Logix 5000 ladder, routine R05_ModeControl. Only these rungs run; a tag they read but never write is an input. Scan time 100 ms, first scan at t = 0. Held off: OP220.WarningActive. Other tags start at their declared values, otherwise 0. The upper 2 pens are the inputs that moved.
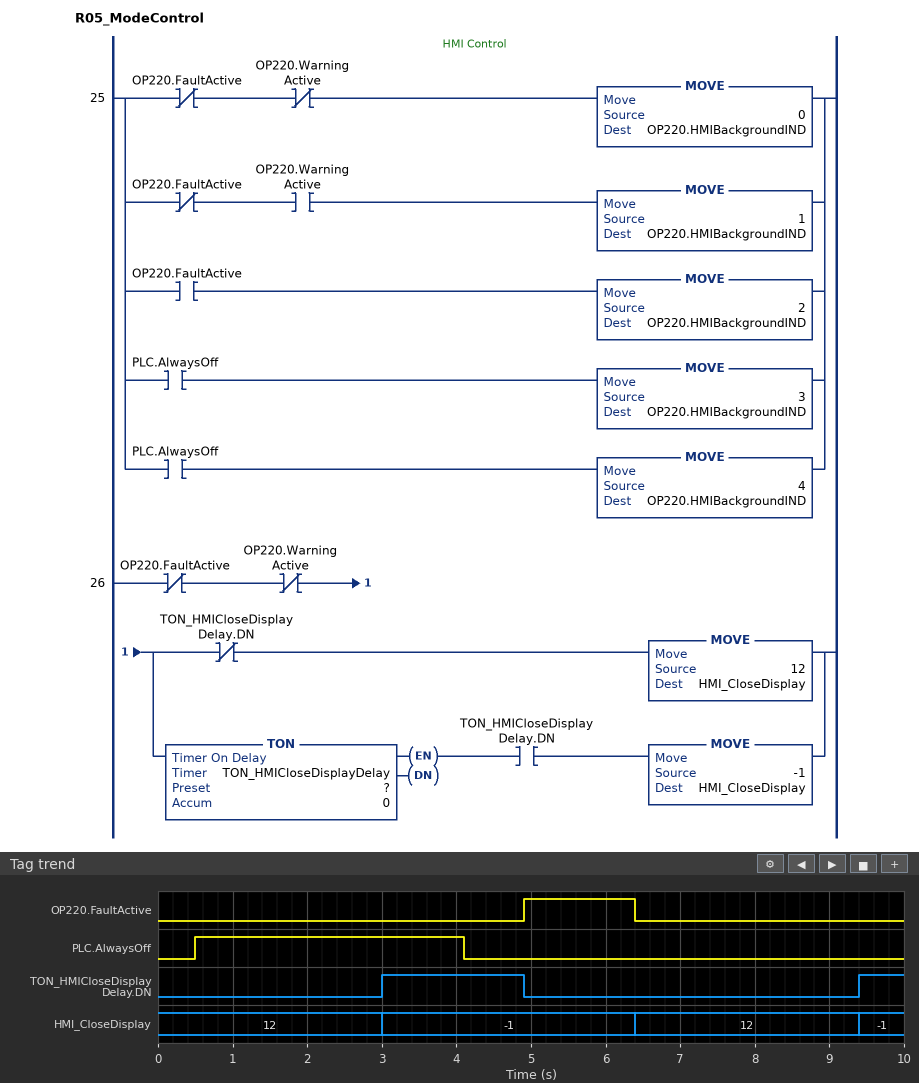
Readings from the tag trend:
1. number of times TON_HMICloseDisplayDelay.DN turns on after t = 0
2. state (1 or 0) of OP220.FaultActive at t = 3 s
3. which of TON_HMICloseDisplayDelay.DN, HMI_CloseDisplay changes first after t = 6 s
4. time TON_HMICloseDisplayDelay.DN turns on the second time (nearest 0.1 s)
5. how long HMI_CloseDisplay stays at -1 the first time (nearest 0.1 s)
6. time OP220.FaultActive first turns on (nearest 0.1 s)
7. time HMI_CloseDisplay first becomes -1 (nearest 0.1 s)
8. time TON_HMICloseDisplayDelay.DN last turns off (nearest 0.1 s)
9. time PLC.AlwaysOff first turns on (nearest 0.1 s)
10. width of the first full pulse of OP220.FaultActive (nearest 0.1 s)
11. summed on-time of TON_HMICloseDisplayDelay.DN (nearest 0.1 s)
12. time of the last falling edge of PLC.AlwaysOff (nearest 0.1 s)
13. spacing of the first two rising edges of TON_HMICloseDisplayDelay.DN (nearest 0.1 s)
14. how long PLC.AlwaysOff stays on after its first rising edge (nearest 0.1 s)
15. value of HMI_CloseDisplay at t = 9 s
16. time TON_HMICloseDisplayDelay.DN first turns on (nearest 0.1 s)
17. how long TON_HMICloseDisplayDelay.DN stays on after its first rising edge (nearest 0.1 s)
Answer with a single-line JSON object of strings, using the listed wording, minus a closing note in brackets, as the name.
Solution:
{"number of times TON_HMICloseDisplayDelay.DN turns on after t = 0": "2", "state (1 or 0) of OP220.FaultActive at t = 3 s": "0", "which of TON_HMICloseDisplayDelay.DN, HMI_CloseDisplay changes first after t = 6 s": "HMI_CloseDisplay", "time TON_HMICloseDisplayDelay.DN turns on the second time": "9.4 s", "how long HMI_CloseDisplay stays at -1 the first time": "3.4 s", "time OP220.FaultActive first turns on": "4.9 s", "time HMI_CloseDisplay first becomes -1": "3.0 s", "time TON_HMICloseDisplayDelay.DN last turns off": "4.9 s", "time PLC.AlwaysOff first turns on": "0.5 s", "width of the first full pulse of OP220.FaultActive": "1.5 s", "summed on-time of TON_HMICloseDisplayDelay.DN": "2.5 s", "time of the last falling edge of PLC.AlwaysOff": "4.1 s", "spacing of the first two rising edges of TON_HMICloseDisplayDelay.DN": "6.4 s", "how long PLC.AlwaysOff stays on after its first rising edge": "3.6 s", "value of HMI_CloseDisplay at t = 9 s": "12", "time TON_HMICloseDisplayDelay.DN first turns on": "3.0 s", "how long TON_HMICloseDisplayDelay.DN stays on after its first rising edge": "1.9 s"}
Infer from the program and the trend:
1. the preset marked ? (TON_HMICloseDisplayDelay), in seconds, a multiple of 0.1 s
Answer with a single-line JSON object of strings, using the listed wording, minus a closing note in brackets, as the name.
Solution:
{"the preset marked ? (TON_HMICloseDisplayDelay), in seconds, a multiple of 0.1 s": "3.0 s"}
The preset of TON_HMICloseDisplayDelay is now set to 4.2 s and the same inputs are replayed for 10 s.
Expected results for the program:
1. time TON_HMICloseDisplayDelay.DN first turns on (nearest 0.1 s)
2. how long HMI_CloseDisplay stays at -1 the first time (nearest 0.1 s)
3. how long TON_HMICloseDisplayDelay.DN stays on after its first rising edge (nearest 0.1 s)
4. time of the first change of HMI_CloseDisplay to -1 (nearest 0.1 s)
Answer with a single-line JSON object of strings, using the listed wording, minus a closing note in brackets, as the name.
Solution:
{"time TON_HMICloseDisplayDelay.DN first turns on": "4.2 s", "how long HMI_CloseDisplay stays at -1 the first time": "2.2 s", "how long TON_HMICloseDisplayDelay.DN stays on after its first rising edge": "0.7 s", "time of the first change of HMI_CloseDisplay to -1": "4.2 s"}
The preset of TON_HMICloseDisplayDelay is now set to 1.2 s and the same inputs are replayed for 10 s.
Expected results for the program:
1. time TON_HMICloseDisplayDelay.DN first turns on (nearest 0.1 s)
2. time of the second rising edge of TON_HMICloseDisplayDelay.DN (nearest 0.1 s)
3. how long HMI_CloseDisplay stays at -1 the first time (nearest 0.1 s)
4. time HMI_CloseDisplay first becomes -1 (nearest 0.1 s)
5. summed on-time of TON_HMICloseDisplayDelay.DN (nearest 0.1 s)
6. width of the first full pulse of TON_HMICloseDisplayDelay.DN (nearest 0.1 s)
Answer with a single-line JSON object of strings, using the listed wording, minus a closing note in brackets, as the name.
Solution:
{"time TON_HMICloseDisplayDelay.DN first turns on": "1.2 s", "time of the second rising edge of TON_HMICloseDisplayDelay.DN": "7.6 s", "how long HMI_CloseDisplay stays at -1 the first time": "5.2 s", "time HMI_CloseDisplay first becomes -1": "1.2 s", "summed on-time of TON_HMICloseDisplayDelay.DN": "6.1 s", "width of the first full pulse of TON_HMICloseDisplayDelay.DN": "3.7 s"}
